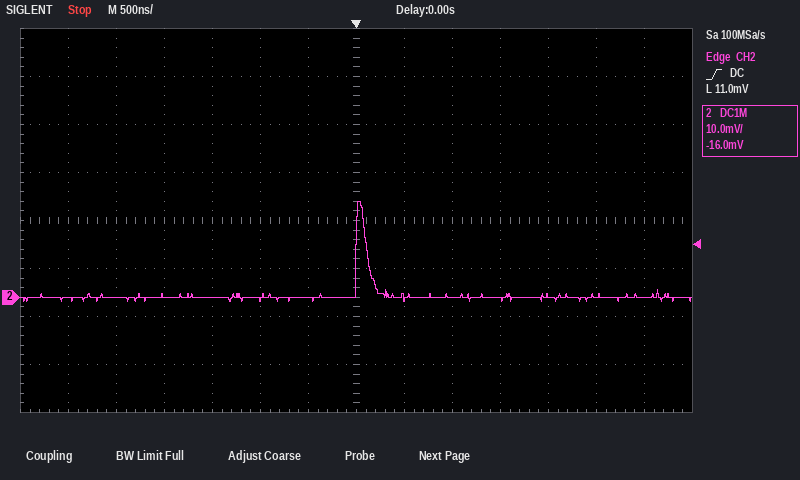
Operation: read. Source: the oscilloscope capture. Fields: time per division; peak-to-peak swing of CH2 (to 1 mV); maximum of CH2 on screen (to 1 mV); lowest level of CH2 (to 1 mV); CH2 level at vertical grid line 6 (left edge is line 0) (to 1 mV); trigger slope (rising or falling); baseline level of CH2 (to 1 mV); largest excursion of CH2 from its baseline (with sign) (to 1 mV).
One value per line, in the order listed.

500 ns
21 mV
20 mV
-1 mV
0 mV
rising
0 mV
+20 mV
